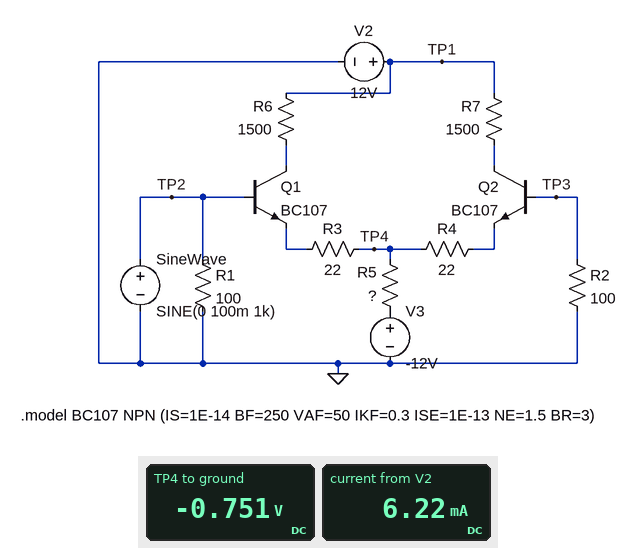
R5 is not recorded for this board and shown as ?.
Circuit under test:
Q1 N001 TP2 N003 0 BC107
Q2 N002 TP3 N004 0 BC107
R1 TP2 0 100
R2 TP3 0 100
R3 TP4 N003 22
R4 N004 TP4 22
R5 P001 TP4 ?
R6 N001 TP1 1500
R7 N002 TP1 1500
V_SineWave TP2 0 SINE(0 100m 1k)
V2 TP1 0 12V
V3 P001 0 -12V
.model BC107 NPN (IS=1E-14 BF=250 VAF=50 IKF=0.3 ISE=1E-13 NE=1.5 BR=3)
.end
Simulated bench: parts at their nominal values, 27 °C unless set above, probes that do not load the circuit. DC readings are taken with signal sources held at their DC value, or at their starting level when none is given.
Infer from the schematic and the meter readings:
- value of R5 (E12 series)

1.8 kΩ
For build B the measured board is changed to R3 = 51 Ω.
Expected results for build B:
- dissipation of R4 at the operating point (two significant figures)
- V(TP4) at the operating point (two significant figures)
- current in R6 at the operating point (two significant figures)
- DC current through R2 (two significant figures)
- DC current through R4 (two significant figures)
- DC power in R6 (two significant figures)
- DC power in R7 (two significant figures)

370 µW
-780 mV
2.1 mA
20 µA
4.1 mA
6.9 mW
25 mW
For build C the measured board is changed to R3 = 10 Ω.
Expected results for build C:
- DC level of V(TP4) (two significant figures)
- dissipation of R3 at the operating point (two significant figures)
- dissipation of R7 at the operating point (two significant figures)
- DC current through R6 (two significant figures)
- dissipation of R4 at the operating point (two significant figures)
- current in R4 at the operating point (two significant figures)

-730 mV
150 µW
8.3 mW
3.9 mA
120 µW
2.4 mA
